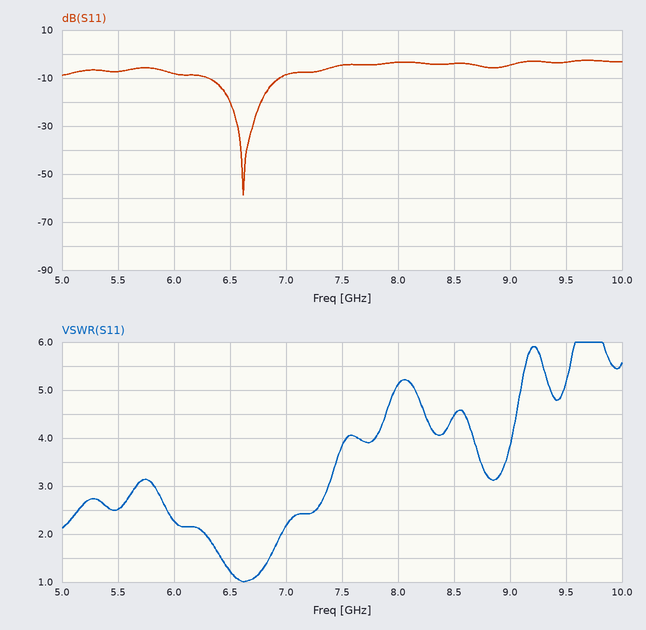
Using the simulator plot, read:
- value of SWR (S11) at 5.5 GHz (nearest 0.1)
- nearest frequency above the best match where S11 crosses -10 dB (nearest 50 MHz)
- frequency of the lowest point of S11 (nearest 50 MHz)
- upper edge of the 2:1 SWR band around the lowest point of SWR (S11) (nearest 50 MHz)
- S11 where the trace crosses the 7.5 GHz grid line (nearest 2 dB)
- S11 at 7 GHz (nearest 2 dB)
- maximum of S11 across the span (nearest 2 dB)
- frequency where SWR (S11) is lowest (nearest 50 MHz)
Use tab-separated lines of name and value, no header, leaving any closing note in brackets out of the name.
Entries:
value of SWR (S11) at 5.5 GHz	2.5
nearest frequency above the best match where S11 crosses -10 dB	6.95 GHz
frequency of the lowest point of S11	6.60 GHz
upper edge of the 2:1 SWR band around the lowest point of SWR (S11)	6.95 GHz
S11 where the trace crosses the 7.5 GHz grid line	-4 dB
S11 at 7 GHz	-8 dB
maximum of S11 across the span	-2 dB
frequency where SWR (S11) is lowest	6.60 GHz
